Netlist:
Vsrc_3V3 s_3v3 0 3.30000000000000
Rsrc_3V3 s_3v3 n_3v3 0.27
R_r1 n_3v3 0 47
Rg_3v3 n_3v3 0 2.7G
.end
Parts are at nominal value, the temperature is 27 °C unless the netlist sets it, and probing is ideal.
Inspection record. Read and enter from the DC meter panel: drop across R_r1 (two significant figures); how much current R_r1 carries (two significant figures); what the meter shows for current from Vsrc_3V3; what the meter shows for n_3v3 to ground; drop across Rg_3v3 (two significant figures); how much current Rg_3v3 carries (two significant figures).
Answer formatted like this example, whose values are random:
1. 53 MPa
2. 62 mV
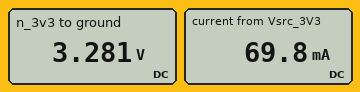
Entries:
1. 3.3 V
2. 70 mA
3. 69.8 mA
4. 3.281 V
5. 3.3 V
6. 1.2 nA
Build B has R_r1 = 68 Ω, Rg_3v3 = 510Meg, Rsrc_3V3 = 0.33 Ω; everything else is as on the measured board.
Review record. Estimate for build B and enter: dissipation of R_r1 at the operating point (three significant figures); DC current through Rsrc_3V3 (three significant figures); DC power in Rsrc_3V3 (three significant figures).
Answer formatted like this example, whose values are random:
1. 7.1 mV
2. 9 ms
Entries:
1. 159 mW
2. 48.3 mA
3. 770 µW
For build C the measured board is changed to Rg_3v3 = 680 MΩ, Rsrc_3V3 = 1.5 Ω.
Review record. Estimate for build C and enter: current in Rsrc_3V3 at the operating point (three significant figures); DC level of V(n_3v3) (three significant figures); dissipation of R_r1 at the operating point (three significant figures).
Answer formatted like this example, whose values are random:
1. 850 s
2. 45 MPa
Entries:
1. 68.0 mA
2. 3.20 V
3. 218 mW
